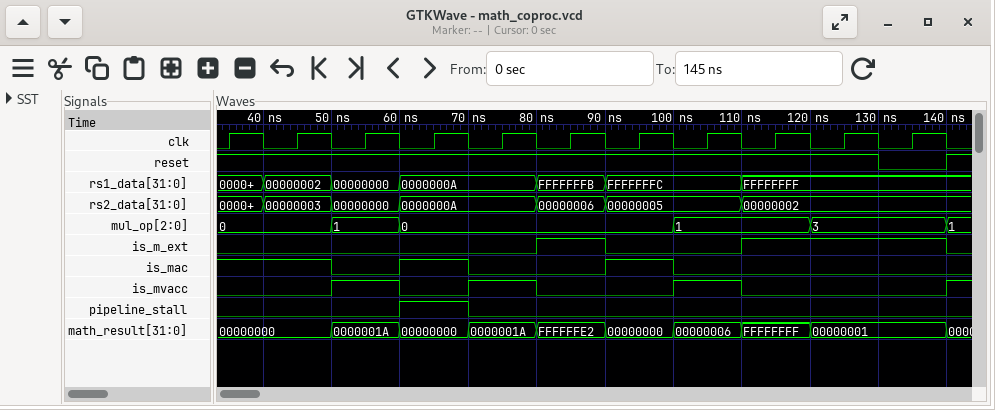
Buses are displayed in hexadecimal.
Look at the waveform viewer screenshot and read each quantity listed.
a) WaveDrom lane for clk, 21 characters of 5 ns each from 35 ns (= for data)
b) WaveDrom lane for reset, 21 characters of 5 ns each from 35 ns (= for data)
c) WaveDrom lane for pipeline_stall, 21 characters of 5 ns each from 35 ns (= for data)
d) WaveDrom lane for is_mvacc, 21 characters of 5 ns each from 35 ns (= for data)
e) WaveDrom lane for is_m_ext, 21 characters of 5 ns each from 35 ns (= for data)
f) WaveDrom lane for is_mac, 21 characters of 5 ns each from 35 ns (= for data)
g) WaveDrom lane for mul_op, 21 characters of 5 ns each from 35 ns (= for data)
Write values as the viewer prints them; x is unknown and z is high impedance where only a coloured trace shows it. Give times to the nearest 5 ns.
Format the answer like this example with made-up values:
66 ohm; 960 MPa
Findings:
{name: 'clk', wave: '101010101010101010101'}; {name: 'reset', wave: '1..................0.'}; {name: 'pipeline_stall', wave: '0....1.0.............'}; {name: 'is_mvacc', wave: '0..1.0.1.0...1.0.....'}; {name: 'is_m_ext', wave: '0........1.0...1.....'}; {name: 'is_mac', wave: '1..0.1.0...1.0.......'}; {name: 'mul_op', wave: '=..=.=.......=...=...', data: '0 1 0 1 3'}
